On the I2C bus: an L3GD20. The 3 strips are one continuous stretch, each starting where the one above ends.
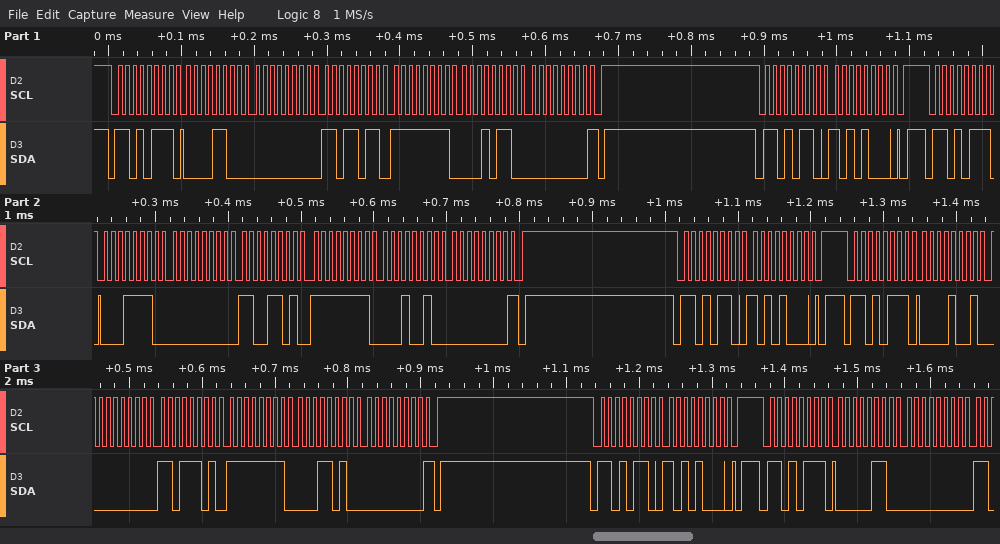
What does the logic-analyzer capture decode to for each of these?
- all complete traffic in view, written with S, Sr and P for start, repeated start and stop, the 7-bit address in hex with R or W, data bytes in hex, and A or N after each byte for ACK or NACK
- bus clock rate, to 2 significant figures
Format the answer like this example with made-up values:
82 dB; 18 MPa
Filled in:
S 6BR A 0C A 00 A DB A FF A 16 A 00 N P S 6BW A A8 A P S 6BR A 1E A 00 A CD A FF A 12 A 00 N P S 6BW A A8 A P S 6BR A 09 A 00 A DD A FF A 1A A 00 N P S 6BW A A8 A P S 6BR A 06 A 00 A; 100 kHz
